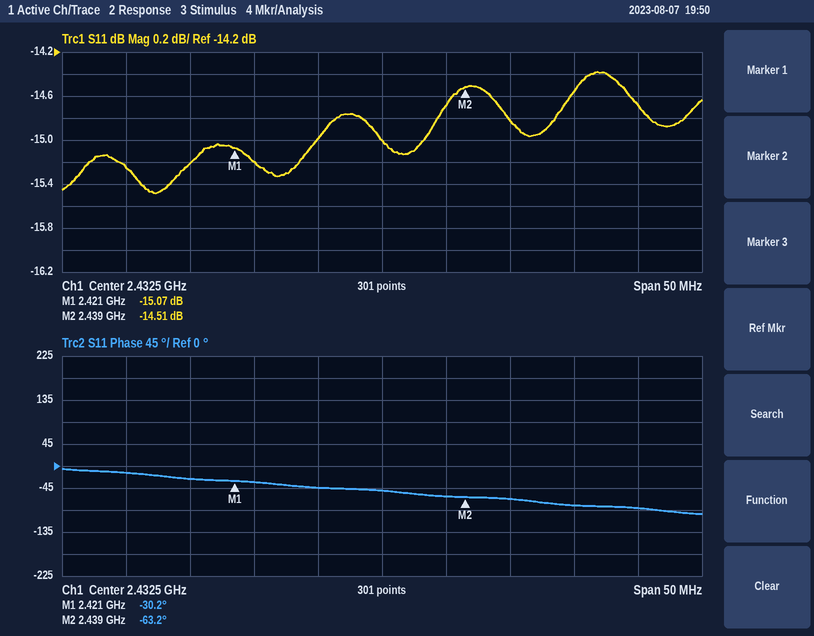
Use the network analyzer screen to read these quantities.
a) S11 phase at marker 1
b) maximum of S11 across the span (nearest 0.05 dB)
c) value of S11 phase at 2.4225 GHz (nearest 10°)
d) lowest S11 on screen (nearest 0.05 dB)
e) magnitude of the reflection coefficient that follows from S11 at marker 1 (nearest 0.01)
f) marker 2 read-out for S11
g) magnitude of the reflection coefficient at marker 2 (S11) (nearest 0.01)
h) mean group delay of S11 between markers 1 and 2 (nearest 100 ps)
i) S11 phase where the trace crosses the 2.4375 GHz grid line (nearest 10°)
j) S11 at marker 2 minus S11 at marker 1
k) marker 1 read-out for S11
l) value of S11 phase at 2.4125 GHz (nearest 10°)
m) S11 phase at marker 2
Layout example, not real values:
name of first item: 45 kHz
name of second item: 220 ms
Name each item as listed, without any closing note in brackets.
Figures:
S11 phase at marker 1: -30.2°
maximum of S11 across the span: -14.40 dB
value of S11 phase at 2.4225 GHz: -30°
lowest S11 on screen: -15.50 dB
magnitude of the reflection coefficient that follows from S11 at marker 1: 0.18
marker 2 read-out for S11: -14.51 dB
magnitude of the reflection coefficient at marker 2 (S11): 0.19
mean group delay of S11 between markers 1 and 2: 5.1 ns
S11 phase where the trace crosses the 2.4375 GHz grid line: -60°
S11 at marker 2 minus S11 at marker 1: 0.56 dB
marker 1 read-out for S11: -15.07 dB
value of S11 phase at 2.4125 GHz: -10°
S11 phase at marker 2: -63.2°
